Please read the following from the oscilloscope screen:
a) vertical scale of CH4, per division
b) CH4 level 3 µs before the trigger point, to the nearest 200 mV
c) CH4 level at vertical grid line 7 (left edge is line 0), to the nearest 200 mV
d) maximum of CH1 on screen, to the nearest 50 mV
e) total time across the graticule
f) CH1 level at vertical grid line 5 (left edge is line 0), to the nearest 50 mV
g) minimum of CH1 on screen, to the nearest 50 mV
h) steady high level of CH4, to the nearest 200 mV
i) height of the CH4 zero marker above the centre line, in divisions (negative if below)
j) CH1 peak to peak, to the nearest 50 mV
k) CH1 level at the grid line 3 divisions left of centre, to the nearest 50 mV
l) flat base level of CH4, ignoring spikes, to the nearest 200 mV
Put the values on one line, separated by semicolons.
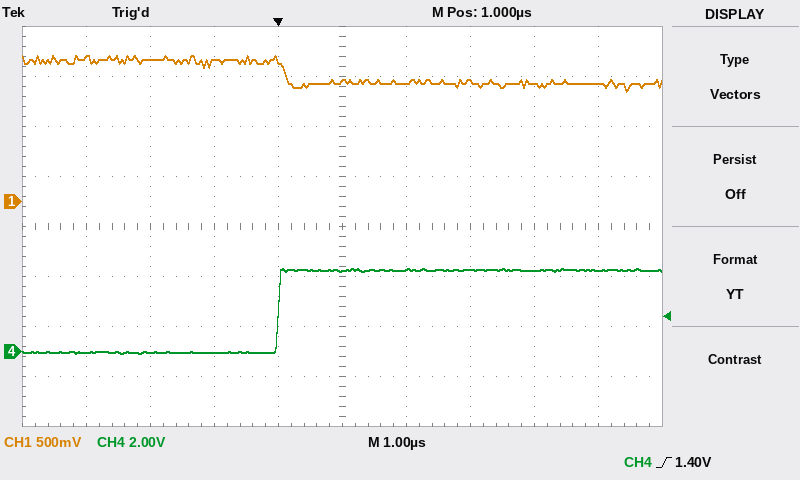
2 V; 0.0 V; 3.2 V; 1.45 V; 10 µs; 1.20 V; 1.10 V; 3.2 V; -2.5 div; 350 mV; 1.40 V; 0.0 V
